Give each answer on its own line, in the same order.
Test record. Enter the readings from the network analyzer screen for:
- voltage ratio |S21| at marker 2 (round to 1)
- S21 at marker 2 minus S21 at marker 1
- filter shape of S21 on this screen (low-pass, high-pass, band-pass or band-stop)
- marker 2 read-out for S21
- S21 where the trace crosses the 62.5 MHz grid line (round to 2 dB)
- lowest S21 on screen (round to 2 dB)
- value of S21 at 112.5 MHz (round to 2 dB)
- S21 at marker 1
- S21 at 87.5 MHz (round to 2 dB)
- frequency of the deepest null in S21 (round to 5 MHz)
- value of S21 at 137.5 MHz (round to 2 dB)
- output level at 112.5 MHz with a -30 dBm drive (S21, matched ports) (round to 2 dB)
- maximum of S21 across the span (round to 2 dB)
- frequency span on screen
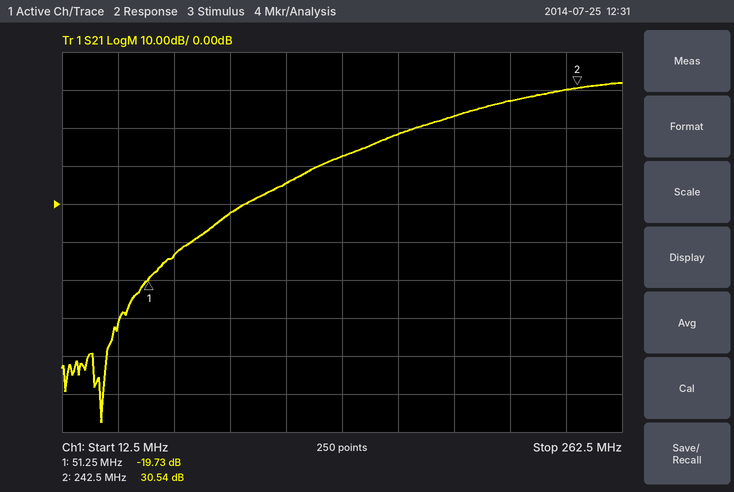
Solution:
34
50.27 dB
high-pass
30.54 dB
-14 dB
-58 dB
6 dB
-19.73 dB
-2 dB
30 MHz
12 dB
-24 dBm
32 dB
250 MHz
